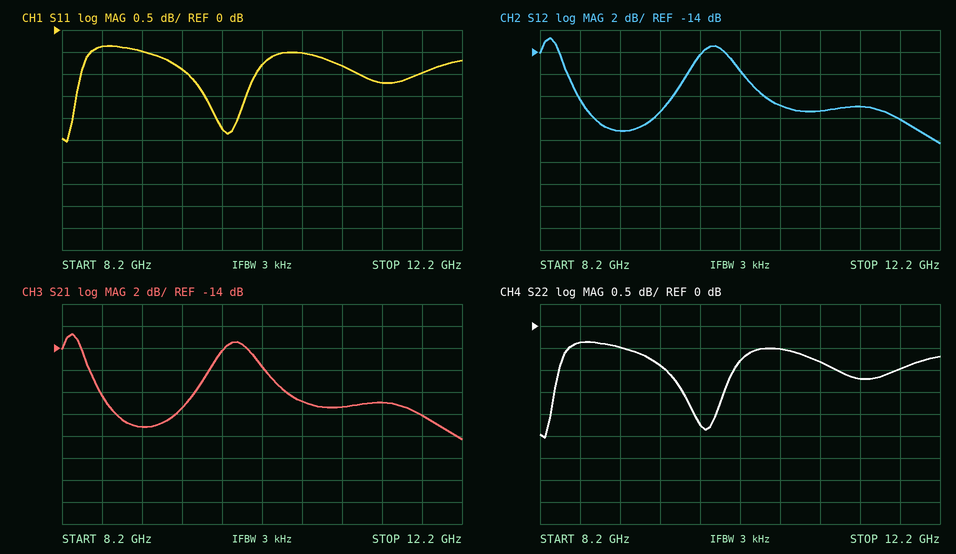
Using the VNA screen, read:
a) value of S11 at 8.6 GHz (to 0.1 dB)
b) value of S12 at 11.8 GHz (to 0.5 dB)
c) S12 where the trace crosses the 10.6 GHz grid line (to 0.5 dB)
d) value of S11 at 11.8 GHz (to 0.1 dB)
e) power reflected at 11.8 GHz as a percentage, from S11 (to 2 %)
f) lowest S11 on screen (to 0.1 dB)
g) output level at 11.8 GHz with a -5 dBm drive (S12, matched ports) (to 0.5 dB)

-0.4 dB
-20.0 dB
-19.0 dB
-1.0 dB
80 %
-2.5 dB
-25.0 dBm
